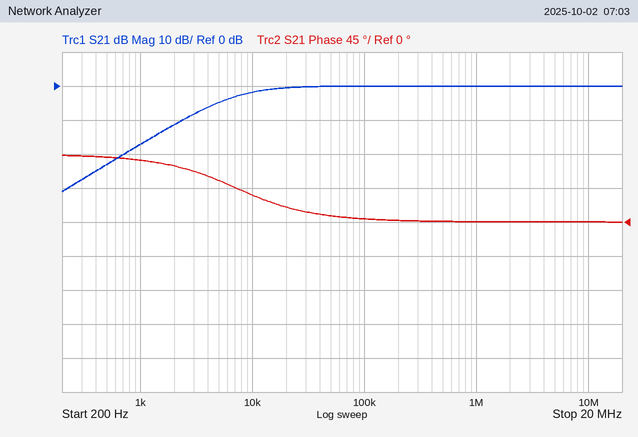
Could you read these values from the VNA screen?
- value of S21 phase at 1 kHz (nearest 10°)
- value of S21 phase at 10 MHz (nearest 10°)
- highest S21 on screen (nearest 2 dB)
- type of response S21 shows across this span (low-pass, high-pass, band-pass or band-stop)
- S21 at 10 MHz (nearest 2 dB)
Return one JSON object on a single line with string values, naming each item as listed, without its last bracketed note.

{"value of S21 phase at 1 kHz": "80°", "value of S21 phase at 10 MHz": "0°", "highest S21 on screen": "0 dB", "type of response S21 shows across this span": "high-pass", "S21 at 10 MHz": "0 dB"}
